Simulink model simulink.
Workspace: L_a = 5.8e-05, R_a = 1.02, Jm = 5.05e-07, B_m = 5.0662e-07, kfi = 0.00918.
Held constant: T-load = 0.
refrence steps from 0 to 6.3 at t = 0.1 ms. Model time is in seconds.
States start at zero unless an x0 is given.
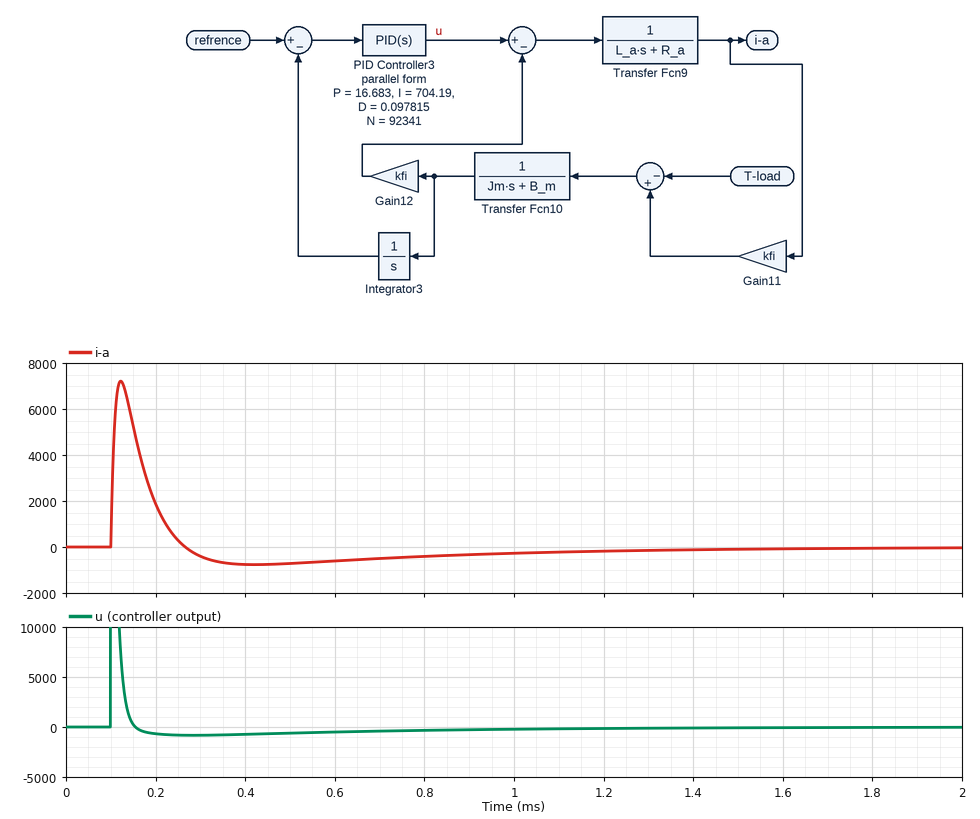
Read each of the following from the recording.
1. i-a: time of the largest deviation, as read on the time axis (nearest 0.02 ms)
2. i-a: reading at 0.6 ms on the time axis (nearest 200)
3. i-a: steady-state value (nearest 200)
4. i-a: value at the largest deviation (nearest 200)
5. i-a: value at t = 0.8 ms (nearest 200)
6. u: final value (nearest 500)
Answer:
0.12 ms
-600
0
7200
-400
0
